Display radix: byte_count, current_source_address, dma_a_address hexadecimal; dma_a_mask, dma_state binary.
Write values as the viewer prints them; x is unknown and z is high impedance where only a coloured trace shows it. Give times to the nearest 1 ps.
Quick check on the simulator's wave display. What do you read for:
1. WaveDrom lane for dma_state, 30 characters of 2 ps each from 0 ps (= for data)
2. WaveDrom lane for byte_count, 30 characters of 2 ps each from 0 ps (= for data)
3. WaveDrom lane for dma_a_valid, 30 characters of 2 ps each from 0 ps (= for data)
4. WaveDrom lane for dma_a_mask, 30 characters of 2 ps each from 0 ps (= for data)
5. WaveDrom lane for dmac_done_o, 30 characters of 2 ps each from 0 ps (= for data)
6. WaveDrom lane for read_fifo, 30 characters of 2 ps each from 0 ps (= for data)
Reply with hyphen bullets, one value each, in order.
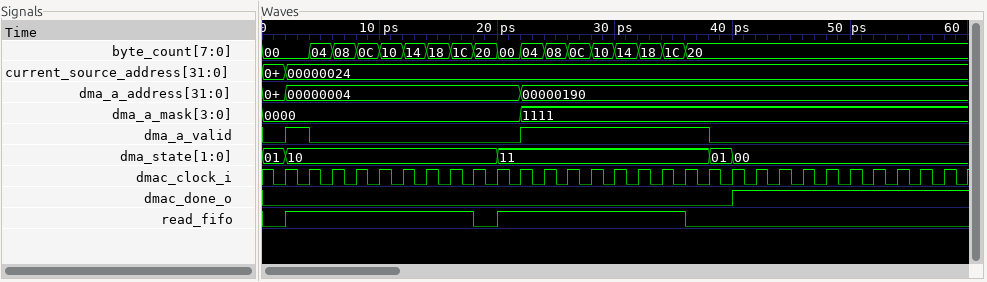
- {name: 'dma_state', wave: '==........=........==.........', data: '01 10 11 01 00'}
- {name: 'byte_count', wave: '=.=================...........', data: '00 04 08 0C 10 14 18 1C 20 00 04 08 0C 10 14 18 1C 20'}
- {name: 'dma_a_valid', wave: '010........1.......0..........'}
- {name: 'dma_a_mask', wave: '=..........=..................', data: '0000 1111'}
- {name: 'dmac_done_o', wave: '0...................1.........'}
- {name: 'read_fifo', wave: '01.......01.......0...........'}
